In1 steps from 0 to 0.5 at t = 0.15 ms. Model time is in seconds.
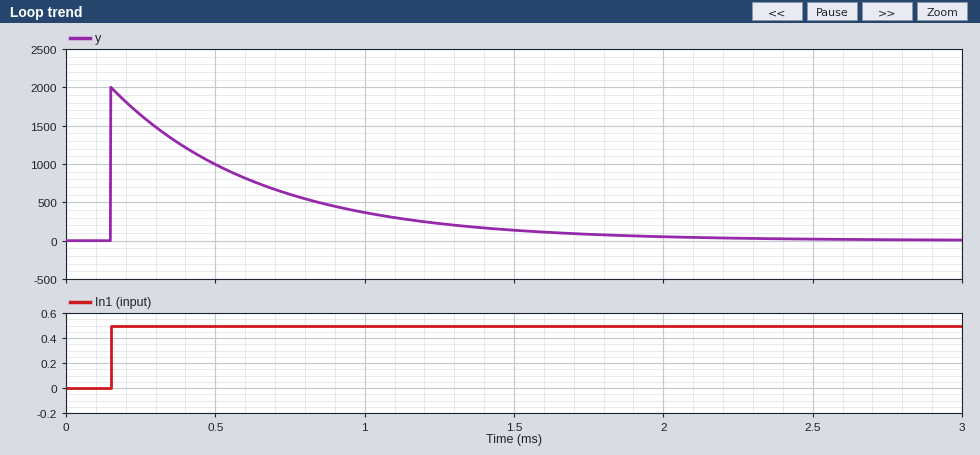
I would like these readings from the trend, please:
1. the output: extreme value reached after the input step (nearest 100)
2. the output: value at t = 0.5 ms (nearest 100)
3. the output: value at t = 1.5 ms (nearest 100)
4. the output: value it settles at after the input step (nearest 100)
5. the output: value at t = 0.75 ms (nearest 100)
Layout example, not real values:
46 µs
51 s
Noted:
2000
1000
100
0
600
